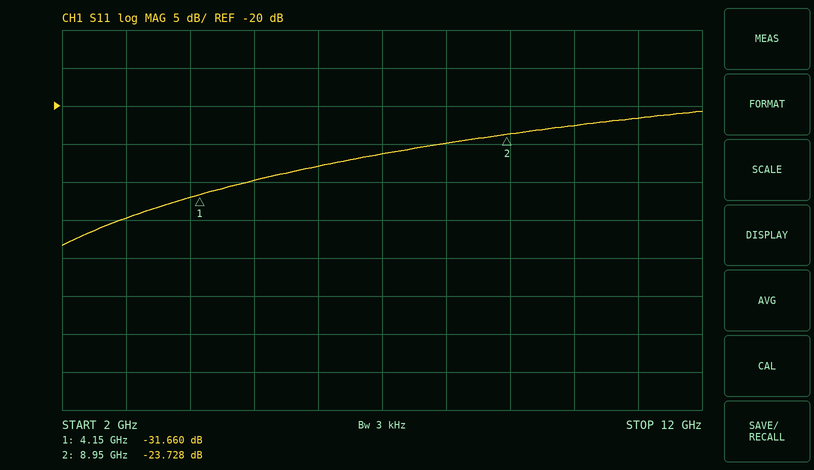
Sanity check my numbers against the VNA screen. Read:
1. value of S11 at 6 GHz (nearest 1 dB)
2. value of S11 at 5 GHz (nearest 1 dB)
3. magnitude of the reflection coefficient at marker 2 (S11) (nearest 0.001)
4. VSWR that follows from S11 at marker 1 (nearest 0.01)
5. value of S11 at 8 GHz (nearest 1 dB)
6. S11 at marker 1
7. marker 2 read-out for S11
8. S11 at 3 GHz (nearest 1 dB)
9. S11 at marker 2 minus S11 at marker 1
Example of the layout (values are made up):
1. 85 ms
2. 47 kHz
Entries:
1. -28 dB
2. -30 dB
3. 0.065
4. 1.05
5. -25 dB
6. -31.660 dB
7. -23.728 dB
8. -35 dB
9. 7.932 dB
